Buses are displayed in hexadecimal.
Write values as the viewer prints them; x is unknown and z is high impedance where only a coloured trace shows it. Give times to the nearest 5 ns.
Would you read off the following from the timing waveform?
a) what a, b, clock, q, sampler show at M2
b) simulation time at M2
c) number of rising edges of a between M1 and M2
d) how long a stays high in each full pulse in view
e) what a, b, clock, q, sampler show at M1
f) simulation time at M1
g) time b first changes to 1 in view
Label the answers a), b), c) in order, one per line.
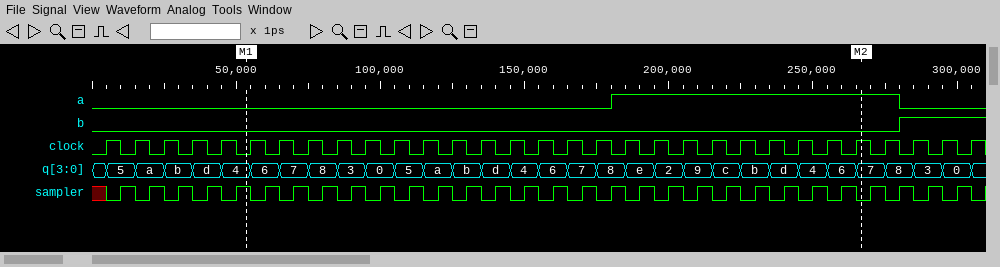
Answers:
a) a=1, b=0, clock=1, q=7, sampler=0
b) 265 ns
c) 1
d) 100 ns
e) a=0, b=0, clock=0, q=4, sampler=1
f) 55 ns
g) 280 ns
